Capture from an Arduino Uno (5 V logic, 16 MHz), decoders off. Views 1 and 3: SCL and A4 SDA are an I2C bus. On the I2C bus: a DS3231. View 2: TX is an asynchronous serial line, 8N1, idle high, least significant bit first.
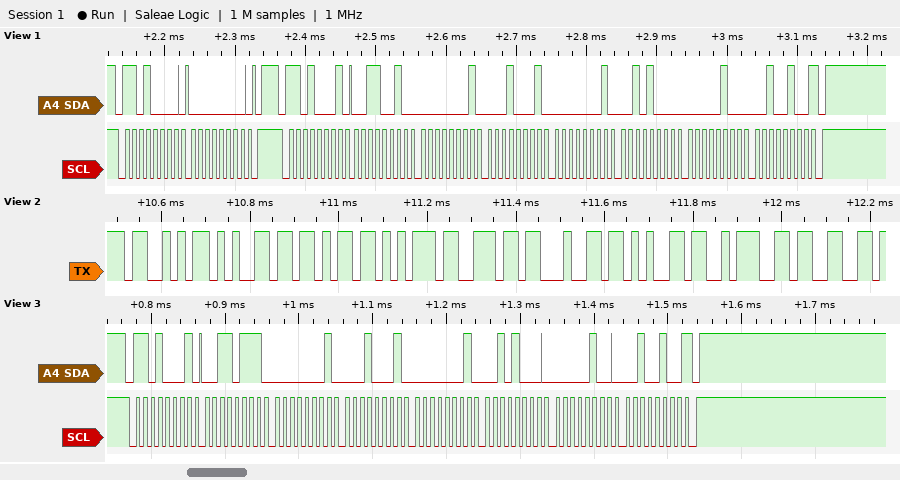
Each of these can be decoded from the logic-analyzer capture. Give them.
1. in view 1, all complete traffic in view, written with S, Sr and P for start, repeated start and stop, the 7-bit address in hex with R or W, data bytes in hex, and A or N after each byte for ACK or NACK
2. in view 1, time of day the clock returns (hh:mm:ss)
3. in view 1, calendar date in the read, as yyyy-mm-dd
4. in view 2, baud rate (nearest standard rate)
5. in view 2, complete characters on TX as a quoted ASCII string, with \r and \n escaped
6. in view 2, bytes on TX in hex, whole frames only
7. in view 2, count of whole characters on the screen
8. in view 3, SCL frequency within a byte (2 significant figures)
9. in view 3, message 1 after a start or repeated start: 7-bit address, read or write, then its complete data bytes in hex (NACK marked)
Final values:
S 68W A 00 A P S 68R A 32 A 01 A 11 A 01 A 28 A 04 A 24 N P
11:01:32
2024-04-28
57600 baud
"Sekunde:3"
53 65 6B 75 6E 64 65 3A 33
9
100 kHz
0x68 read: 37 01 11 01 28 04 24 NACK
